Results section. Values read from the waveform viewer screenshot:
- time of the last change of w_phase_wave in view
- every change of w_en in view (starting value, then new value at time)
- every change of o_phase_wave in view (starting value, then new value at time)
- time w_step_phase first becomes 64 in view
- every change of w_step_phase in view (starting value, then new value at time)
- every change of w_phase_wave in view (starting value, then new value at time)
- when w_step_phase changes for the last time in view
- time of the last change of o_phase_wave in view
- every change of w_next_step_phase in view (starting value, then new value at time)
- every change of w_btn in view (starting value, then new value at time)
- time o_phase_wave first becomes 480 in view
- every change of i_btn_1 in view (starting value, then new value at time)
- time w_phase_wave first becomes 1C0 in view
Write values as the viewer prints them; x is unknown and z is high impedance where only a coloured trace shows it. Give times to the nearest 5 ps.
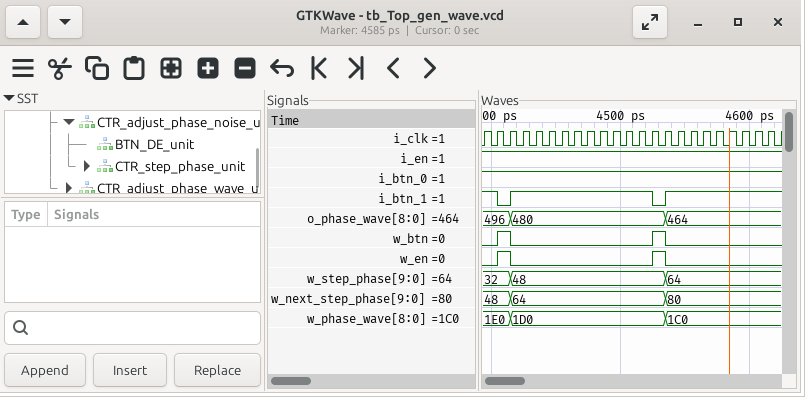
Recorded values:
4535 ps
0, 1 at 4405 ps, 0 at 4415 ps, 1 at 4525 ps, 0 at 4535 ps
496, 480 at 4415 ps, 464 at 4535 ps
4535 ps
32, 48 at 4415 ps, 64 at 4535 ps
1E0, 1D0 at 4415 ps, 1C0 at 4535 ps
4535 ps
4535 ps
48, 64 at 4415 ps, 80 at 4535 ps
0, 1 at 4405 ps, 0 at 4415 ps, 1 at 4525 ps, 0 at 4535 ps
4415 ps
1, 0 at 4405 ps, 1 at 4415 ps, 0 at 4525 ps, 1 at 4535 ps
4535 ps
